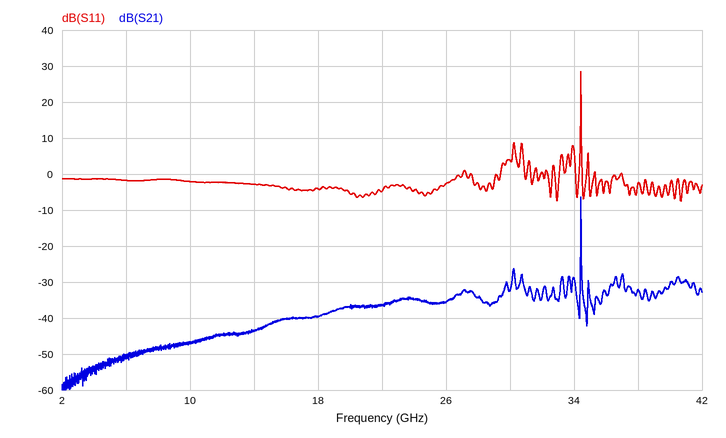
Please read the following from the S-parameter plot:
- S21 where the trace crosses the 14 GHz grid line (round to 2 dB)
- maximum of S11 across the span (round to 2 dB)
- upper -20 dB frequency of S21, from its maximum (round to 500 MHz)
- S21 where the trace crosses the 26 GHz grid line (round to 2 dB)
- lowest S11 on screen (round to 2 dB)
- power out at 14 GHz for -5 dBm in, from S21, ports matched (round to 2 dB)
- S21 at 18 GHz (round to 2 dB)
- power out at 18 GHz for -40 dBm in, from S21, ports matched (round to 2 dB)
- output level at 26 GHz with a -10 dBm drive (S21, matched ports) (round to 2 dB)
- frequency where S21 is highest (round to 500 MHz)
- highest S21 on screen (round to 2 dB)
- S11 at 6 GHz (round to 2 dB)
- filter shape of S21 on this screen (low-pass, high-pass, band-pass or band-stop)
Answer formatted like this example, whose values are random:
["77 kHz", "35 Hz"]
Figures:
["-44 dB", "28 dB", "34.5 GHz", "-36 dB", "-8 dB", "-48 dBm", "-40 dB", "-80 dBm", "-46 dBm", "34.5 GHz", "-6 dB", "-2 dB", "band-pass"]
